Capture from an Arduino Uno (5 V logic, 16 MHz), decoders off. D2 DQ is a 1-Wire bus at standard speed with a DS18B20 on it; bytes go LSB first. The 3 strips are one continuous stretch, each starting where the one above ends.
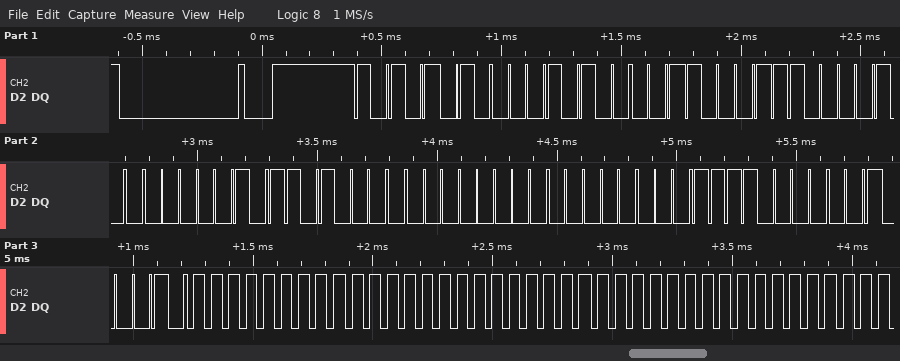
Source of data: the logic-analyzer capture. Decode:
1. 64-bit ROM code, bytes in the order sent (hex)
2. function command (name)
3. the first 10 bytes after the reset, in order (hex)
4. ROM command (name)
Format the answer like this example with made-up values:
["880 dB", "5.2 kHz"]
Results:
["28 8C 43 40 0B 00 00 0F", "Convert T", "55 28 8C 43 40 0B 00 00 0F 44", "Match ROM"]
